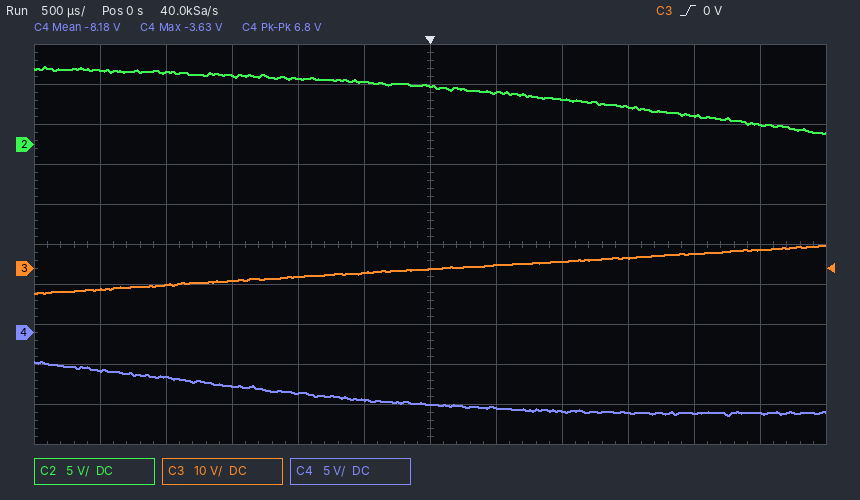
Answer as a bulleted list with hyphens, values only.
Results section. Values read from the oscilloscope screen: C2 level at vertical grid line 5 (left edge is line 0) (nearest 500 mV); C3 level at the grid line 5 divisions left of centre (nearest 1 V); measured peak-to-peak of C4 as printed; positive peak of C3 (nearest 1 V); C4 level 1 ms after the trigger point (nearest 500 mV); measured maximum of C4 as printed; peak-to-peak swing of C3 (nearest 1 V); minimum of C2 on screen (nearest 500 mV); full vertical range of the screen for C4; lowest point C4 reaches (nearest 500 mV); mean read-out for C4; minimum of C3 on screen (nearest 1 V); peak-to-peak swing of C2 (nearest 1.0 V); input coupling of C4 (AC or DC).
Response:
- 8.0 V
- -5 V
- 6.8 V
- 6 V
- -10.0 V
- -3.63 V
- 12 V
- 1.5 V
- 50 V
- -10.5 V
- -8.18 V
- -6 V
- 8.0 V
- DC
